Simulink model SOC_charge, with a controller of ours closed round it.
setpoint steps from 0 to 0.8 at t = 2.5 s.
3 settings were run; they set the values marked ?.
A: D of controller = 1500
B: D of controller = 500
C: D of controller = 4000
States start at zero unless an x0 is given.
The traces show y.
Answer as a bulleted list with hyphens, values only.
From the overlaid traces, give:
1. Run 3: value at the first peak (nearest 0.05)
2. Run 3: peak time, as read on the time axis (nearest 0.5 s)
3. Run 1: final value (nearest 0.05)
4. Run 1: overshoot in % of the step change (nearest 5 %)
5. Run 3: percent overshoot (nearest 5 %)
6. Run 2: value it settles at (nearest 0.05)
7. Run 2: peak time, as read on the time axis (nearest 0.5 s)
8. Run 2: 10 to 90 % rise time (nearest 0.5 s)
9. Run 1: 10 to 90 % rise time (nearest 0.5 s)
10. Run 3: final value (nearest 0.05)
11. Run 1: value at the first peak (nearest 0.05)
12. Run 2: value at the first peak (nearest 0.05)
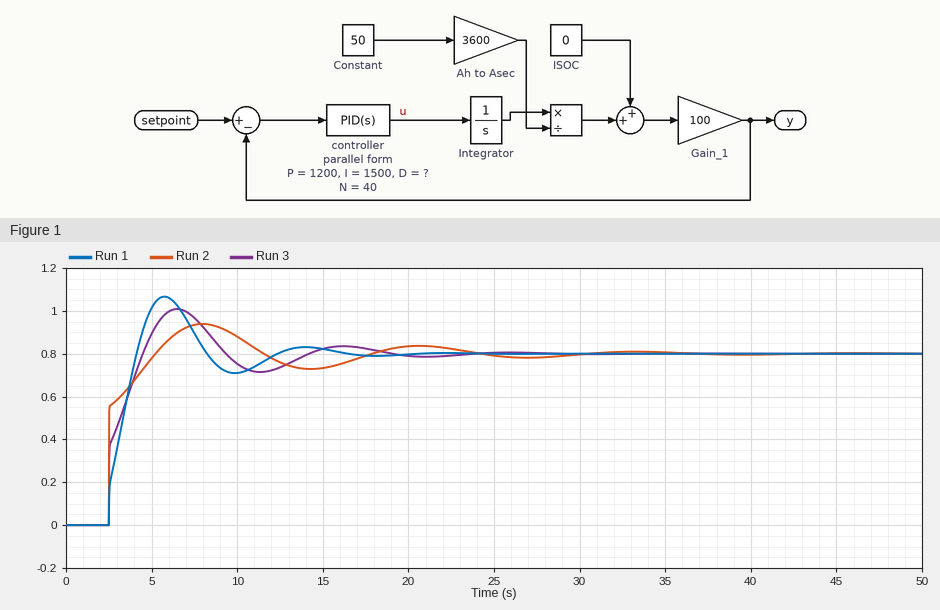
- 1.00
- 6.5 s
- 0.80
- 35 %
- 25 %
- 0.80
- 8.0 s
- 2.0 s
- 1.5 s
- 0.80
- 1.05
- 0.95
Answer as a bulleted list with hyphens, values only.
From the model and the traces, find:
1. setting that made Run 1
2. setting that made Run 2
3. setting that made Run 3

- B
- C
- A
